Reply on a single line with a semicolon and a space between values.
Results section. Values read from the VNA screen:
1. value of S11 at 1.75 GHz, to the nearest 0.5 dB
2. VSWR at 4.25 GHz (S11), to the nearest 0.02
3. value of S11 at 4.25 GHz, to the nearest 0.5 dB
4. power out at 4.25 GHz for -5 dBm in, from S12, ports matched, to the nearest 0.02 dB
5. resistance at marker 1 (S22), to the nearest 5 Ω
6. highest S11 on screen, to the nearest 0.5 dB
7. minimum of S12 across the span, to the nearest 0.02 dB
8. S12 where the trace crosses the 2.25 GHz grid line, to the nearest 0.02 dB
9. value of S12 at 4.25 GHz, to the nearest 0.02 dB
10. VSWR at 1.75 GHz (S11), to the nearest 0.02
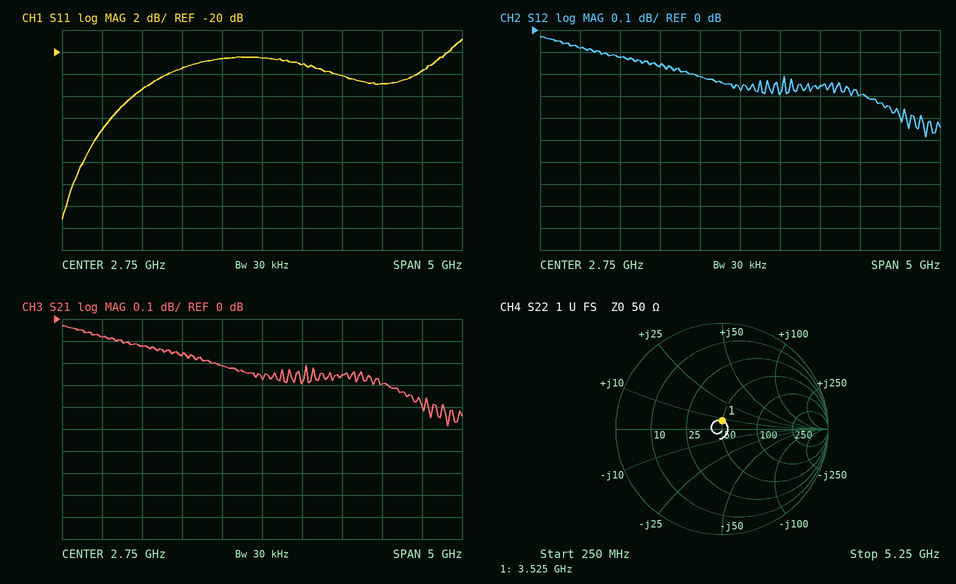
-21.5 dB; 1.16; -23.0 dB; -5.30 dBm; 50 Ω; -19.0 dB; -0.48 dB; -0.22 dB; -0.30 dB; 1.18
